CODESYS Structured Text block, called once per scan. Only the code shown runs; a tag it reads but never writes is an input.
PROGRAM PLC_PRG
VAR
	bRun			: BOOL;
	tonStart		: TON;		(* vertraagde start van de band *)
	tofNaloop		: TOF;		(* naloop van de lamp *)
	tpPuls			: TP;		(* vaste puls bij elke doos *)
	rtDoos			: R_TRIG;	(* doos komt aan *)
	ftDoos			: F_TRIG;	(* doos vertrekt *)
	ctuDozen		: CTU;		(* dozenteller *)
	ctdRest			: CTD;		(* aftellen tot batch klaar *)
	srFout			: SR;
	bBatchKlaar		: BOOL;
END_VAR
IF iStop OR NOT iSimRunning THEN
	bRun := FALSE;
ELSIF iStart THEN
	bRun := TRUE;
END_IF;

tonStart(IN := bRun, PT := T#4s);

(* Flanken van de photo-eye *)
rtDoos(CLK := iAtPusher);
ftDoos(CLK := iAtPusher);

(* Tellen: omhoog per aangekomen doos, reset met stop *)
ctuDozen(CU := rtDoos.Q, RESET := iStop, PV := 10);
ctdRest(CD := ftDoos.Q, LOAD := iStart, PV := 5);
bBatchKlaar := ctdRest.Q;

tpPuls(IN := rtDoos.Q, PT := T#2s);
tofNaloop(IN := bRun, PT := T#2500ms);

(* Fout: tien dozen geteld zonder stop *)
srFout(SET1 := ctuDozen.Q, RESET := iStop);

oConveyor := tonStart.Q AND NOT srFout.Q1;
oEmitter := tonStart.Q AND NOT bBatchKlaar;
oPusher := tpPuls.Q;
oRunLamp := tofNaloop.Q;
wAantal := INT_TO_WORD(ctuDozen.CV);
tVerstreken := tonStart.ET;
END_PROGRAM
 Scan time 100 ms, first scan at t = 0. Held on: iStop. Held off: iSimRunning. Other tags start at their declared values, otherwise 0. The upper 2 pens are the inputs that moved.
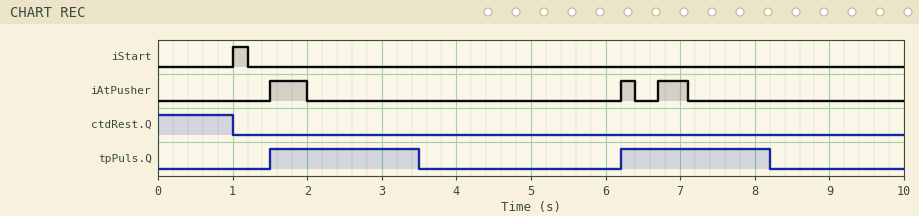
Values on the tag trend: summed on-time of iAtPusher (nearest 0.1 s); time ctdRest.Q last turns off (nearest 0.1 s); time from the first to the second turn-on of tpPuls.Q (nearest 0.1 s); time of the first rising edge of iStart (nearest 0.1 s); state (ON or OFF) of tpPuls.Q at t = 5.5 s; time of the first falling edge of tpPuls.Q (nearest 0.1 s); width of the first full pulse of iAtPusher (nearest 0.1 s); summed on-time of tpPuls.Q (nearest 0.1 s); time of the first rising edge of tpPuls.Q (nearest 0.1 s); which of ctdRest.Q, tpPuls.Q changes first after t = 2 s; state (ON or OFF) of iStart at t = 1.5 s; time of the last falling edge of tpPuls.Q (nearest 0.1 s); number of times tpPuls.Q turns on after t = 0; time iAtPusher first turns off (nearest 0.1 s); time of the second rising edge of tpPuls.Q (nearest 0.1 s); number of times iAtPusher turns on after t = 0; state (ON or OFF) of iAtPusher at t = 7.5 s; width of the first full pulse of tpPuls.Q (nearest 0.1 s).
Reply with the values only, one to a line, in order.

1.1 s
1.0 s
4.7 s
1.0 s
OFF
3.5 s
0.5 s
4.0 s
1.5 s
tpPuls.Q
OFF
8.2 s
2
2.0 s
6.2 s
3
OFF
2.0 s
